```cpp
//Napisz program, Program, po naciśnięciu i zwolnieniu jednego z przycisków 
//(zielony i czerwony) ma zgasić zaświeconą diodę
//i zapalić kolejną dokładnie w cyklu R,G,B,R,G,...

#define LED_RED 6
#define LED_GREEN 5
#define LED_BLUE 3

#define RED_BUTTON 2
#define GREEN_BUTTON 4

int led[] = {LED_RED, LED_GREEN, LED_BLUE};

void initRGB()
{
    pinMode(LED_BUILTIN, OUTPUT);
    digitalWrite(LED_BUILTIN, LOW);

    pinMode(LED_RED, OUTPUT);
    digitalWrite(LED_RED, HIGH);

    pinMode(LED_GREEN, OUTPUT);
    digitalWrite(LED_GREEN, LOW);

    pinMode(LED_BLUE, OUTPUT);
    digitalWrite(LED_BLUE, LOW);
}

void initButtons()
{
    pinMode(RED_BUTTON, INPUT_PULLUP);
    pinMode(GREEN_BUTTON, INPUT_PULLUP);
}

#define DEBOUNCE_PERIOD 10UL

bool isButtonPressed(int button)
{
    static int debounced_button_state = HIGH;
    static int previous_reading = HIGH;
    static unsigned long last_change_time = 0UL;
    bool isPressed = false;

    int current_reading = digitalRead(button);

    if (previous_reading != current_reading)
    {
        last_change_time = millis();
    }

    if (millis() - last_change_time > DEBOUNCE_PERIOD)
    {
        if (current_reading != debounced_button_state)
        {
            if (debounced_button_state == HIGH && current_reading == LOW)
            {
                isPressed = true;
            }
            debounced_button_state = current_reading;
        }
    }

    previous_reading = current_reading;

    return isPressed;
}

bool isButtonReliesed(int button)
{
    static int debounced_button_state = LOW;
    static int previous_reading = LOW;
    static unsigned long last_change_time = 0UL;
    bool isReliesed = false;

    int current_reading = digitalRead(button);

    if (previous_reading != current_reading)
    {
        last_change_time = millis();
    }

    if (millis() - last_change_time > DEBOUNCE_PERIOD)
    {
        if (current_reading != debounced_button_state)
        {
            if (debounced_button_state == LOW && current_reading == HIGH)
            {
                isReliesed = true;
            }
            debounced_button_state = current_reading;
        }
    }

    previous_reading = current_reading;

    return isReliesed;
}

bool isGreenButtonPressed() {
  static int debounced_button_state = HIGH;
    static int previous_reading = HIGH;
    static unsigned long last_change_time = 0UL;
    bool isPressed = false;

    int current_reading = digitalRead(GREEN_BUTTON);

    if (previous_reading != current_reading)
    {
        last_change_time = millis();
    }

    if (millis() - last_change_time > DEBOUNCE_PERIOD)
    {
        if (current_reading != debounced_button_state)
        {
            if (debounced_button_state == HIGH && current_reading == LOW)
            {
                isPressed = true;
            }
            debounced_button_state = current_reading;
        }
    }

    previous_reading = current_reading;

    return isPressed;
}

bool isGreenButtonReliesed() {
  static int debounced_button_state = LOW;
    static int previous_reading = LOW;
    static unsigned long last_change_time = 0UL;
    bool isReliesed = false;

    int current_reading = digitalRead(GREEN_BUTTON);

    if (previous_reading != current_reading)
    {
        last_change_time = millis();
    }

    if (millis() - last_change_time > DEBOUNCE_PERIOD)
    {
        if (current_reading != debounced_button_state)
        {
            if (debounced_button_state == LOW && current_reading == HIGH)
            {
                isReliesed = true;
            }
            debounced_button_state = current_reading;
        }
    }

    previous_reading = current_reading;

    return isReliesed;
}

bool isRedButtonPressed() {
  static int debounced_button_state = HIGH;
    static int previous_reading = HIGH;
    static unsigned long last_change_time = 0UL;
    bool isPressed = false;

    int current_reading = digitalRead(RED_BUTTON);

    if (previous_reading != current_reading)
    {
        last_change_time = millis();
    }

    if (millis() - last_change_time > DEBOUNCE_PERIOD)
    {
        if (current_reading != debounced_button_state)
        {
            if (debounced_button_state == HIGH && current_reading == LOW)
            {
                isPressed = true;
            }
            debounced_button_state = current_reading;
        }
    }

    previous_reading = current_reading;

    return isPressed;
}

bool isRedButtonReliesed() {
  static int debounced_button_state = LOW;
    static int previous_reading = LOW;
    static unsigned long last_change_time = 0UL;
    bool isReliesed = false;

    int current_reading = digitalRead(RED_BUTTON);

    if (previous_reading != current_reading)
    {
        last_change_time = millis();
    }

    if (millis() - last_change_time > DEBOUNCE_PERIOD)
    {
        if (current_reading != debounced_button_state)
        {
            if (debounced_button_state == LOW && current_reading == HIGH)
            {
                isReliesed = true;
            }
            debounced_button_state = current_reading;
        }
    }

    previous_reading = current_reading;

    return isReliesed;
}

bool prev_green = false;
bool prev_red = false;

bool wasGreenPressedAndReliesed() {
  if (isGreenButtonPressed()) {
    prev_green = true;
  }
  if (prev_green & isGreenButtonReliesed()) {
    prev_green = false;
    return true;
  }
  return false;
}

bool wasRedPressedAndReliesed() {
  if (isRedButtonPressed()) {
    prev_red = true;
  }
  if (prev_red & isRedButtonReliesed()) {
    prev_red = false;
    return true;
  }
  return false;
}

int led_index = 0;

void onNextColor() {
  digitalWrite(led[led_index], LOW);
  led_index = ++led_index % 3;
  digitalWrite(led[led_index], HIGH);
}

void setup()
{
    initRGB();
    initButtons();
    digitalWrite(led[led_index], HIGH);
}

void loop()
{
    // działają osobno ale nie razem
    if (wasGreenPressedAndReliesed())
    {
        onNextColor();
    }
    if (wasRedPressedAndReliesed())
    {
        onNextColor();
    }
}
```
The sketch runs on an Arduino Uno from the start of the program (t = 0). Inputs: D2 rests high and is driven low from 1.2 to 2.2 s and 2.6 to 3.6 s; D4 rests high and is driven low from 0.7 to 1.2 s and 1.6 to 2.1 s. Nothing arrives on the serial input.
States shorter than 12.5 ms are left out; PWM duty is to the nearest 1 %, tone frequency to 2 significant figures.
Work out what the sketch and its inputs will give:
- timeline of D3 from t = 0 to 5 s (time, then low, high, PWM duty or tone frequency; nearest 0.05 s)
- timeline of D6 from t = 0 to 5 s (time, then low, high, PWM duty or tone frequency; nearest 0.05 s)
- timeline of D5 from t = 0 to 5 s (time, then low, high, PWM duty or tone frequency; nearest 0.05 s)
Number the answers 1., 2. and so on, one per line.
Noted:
1. 0 s low; 2.1 s high; 2.2 s low
2. 0 s high; 1.2 s low; 2.2 s high; 3.6 s low
3. 0 s low; 1.2 s high; 2.1 s low; 3.6 s high
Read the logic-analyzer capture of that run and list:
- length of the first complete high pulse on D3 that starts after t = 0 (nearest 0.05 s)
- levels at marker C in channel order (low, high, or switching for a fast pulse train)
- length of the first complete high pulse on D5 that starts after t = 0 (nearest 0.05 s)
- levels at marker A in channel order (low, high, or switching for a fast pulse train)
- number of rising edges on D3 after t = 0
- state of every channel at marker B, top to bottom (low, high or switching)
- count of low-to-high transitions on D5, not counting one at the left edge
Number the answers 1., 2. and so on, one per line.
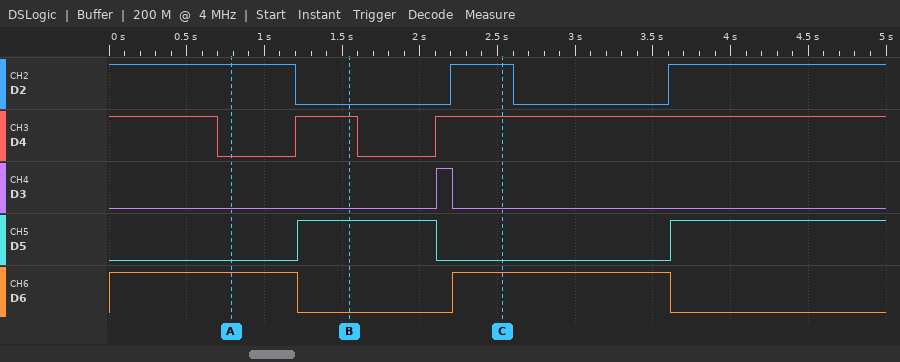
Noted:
1. 0.10 s
2. D2 high, D4 high, D3 low, D5 low, D6 high
3. 0.90 s
4. D2 high, D4 low, D3 low, D5 low, D6 high
5. 1
6. D2 low, D4 high, D3 low, D5 high, D6 low
7. 2
